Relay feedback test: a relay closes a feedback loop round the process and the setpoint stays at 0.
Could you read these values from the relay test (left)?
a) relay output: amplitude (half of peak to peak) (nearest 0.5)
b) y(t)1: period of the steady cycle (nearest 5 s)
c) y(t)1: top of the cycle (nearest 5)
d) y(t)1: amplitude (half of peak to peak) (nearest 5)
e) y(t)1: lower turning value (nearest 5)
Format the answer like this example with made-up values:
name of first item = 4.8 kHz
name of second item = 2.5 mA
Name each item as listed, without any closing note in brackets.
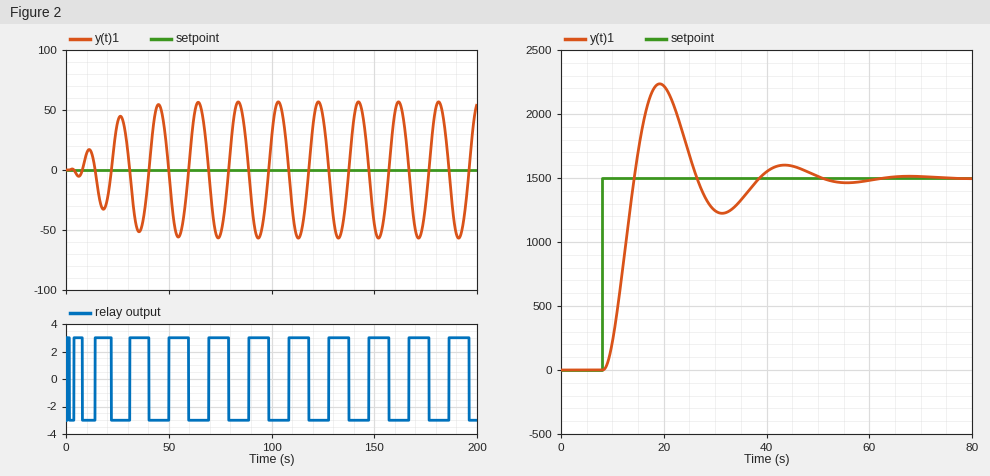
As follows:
relay output: amplitude (half of peak to peak) = 3.0
y(t)1: period of the steady cycle = 20 s
y(t)1: top of the cycle = 55
y(t)1: amplitude (half of peak to peak) = 55
y(t)1: lower turning value = -55
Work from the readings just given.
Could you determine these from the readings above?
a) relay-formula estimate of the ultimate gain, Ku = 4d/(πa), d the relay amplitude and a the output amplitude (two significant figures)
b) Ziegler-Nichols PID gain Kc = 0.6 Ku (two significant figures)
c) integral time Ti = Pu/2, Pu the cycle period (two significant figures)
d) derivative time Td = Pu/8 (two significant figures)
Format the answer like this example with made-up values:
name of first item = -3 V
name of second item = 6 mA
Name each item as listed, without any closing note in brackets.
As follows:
relay-formula estimate of the ultimate gain, Ku = 4d/(πa), d the relay amplitude and a the output amplitude = 0.069
Ziegler-Nichols PID gain Kc = 0.6 Ku = 0.041
integral time Ti = Pu/2, Pu the cycle period = 10 s
derivative time Td = Pu/8 = 2.5 s
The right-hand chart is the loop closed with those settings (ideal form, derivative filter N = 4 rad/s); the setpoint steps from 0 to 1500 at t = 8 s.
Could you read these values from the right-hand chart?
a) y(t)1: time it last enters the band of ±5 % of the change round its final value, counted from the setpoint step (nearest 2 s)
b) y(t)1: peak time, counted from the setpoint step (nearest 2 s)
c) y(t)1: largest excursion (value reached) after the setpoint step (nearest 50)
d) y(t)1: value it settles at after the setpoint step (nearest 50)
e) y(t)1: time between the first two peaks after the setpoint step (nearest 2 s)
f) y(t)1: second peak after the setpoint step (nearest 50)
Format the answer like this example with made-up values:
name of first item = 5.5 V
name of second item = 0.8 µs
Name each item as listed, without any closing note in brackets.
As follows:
y(t)1: time it last enters the band of ±5 % of the change round its final value, counted from the setpoint step = 38 s
y(t)1: peak time, counted from the setpoint step = 12 s
y(t)1: largest excursion (value reached) after the setpoint step = 2250
y(t)1: value it settles at after the setpoint step = 1500
y(t)1: time between the first two peaks after the setpoint step = 24 s
y(t)1: second peak after the setpoint step = 1600
